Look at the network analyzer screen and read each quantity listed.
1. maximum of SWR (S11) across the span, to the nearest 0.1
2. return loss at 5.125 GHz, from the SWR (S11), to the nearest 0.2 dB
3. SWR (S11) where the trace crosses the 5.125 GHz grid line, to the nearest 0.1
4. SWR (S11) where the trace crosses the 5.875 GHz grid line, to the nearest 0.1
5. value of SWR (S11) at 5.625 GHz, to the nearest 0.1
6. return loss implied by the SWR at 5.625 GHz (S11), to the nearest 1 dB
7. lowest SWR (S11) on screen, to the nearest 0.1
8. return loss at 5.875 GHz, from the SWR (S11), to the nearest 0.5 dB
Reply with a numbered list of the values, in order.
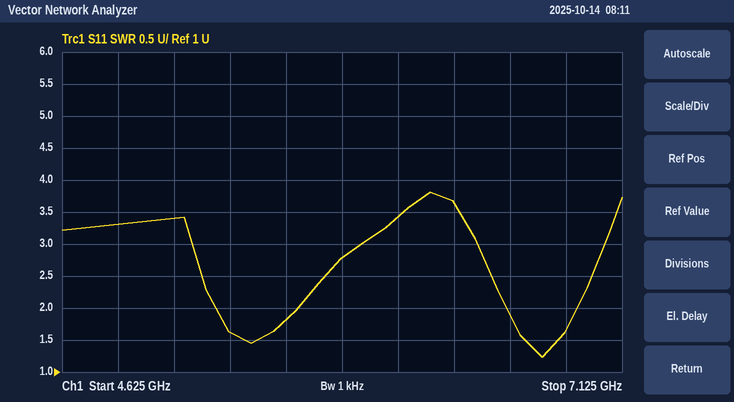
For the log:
1. 3.8
2. 5.2 dB
3. 3.4
4. 2.8
5. 1.8
6. 11 dB
7. 1.2
8. 6.5 dB
